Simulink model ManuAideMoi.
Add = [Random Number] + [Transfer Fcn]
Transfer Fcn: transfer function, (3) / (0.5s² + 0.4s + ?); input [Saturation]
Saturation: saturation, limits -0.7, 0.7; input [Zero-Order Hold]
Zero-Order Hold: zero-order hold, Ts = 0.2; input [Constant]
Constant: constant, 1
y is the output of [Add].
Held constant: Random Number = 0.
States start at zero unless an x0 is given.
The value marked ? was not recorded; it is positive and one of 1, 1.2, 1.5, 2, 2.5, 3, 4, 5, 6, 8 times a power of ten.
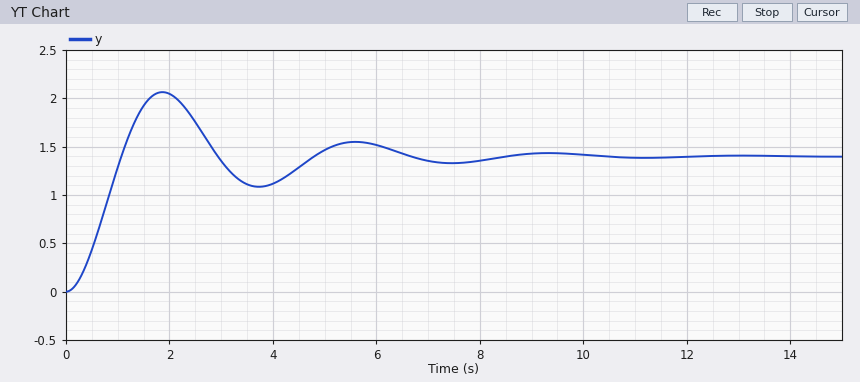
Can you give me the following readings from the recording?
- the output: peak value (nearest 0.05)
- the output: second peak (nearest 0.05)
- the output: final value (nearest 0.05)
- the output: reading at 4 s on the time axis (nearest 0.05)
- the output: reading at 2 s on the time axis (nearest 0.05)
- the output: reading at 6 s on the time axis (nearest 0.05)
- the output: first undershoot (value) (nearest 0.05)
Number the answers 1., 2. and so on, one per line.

1. 2.05
2. 1.55
3. 1.40
4. 1.10
5. 2.05
6. 1.50
7. 1.10
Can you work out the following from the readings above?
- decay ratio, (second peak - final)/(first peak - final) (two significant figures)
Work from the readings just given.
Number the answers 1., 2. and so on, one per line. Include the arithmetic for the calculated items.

1. (1.55 - 1.4) / (2.05 - 1.4) = 0.23
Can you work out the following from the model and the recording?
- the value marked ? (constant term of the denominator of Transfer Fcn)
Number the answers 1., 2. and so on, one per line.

1. 1.5
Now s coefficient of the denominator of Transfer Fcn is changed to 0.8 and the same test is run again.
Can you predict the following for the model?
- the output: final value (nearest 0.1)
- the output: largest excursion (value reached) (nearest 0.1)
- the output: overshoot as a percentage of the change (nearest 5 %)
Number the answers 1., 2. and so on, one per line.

1. 1.4
2. 1.7
3. 20 %
